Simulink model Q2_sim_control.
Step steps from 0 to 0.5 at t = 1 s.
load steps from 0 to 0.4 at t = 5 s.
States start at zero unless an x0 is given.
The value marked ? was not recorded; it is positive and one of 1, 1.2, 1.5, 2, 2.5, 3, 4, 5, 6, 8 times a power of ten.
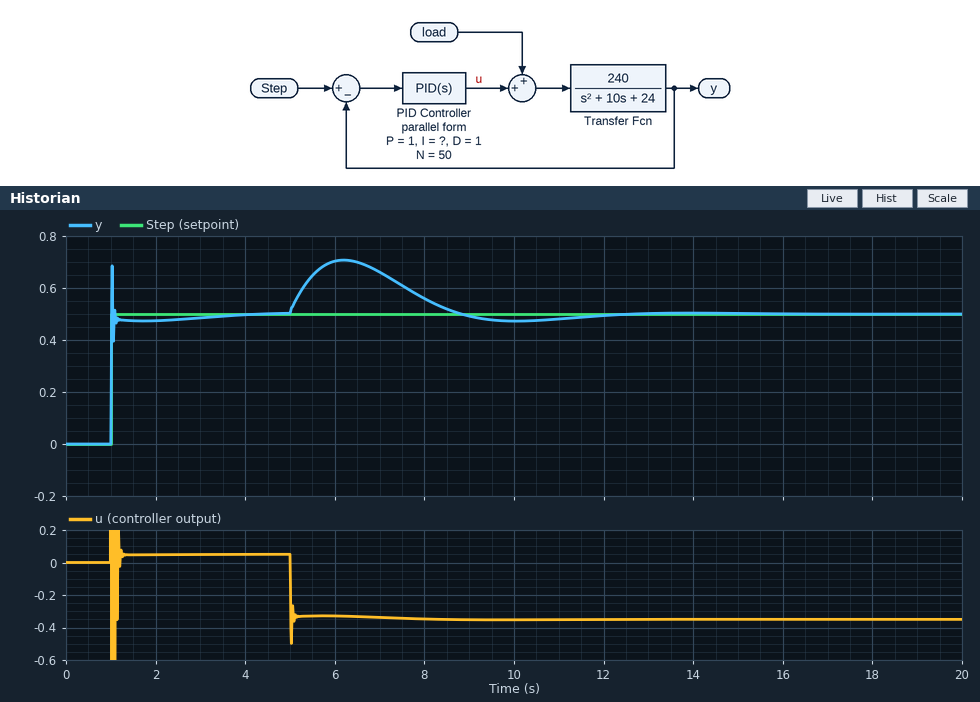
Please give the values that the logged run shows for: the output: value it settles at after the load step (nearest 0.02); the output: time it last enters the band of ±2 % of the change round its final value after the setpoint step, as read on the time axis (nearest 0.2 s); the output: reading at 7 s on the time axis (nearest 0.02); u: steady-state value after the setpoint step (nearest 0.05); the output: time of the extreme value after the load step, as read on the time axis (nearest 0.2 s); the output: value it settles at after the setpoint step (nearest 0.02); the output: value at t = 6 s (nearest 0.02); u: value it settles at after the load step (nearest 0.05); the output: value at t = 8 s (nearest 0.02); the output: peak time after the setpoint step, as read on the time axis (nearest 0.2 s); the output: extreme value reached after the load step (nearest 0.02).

0.50
3.4 s
0.66
0.05
6.2 s
0.50
0.70
-0.35
0.56
1.0 s
0.70
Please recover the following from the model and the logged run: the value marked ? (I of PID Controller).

1
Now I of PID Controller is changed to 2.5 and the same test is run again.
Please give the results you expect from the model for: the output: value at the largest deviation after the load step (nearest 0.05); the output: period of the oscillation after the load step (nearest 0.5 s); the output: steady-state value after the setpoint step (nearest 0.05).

0.65
4.5 s
0.50
